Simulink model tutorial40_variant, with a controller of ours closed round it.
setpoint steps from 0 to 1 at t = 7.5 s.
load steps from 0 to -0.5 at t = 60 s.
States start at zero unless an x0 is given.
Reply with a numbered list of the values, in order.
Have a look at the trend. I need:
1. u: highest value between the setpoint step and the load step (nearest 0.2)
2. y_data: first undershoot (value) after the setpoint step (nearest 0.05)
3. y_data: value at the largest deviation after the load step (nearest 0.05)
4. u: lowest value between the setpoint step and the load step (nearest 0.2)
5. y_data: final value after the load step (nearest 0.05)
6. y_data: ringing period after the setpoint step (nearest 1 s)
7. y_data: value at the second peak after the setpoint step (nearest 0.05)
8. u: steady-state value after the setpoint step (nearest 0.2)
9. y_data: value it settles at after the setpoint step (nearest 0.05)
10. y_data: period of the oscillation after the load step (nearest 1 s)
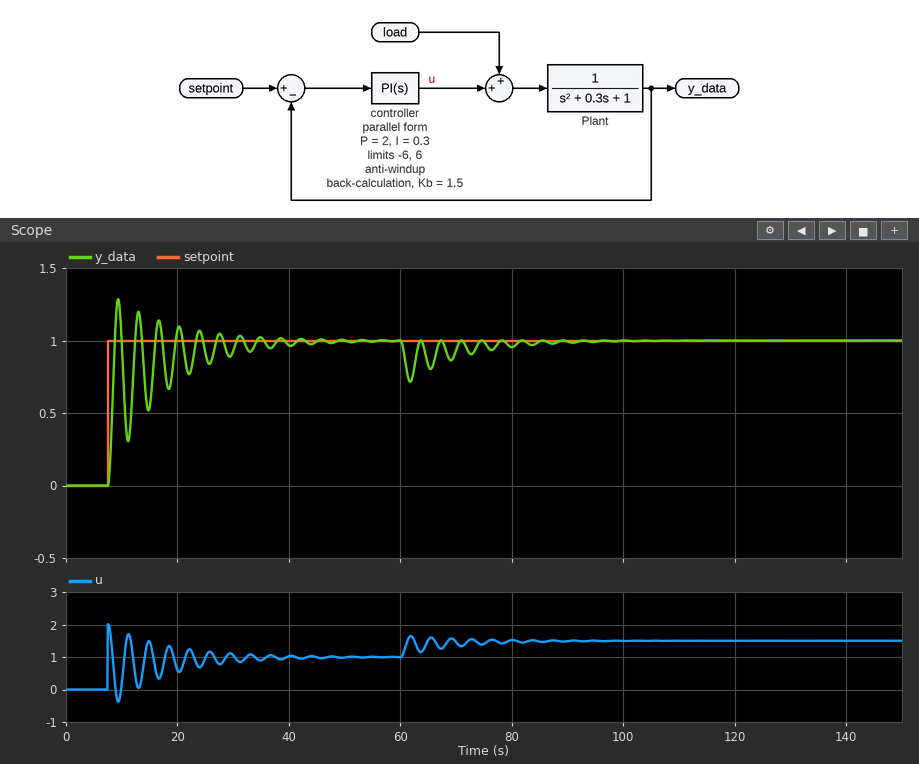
1. 2.0
2. 0.30
3. 0.70
4. -0.4
5. 1.00
6. 4 s
7. 1.20
8. 1.0
9. 1.00
10. 4 s
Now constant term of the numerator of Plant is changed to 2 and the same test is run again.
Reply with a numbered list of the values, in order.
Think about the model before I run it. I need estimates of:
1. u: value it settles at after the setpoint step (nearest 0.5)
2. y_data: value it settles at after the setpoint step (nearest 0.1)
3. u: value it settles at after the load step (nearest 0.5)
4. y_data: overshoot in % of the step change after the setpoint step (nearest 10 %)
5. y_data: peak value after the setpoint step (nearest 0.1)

1. 0.5
2. 1.0
3. 1.0
4. 50 %
5. 1.5
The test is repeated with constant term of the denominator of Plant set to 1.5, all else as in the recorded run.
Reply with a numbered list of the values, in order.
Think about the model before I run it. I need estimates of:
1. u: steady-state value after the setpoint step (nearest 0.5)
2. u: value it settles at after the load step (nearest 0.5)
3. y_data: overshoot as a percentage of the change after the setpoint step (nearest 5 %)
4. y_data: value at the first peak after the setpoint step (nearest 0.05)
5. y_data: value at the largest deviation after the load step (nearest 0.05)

1. 1.5
2. 2.0
3. 10 %
4. 1.10
5. 0.75
